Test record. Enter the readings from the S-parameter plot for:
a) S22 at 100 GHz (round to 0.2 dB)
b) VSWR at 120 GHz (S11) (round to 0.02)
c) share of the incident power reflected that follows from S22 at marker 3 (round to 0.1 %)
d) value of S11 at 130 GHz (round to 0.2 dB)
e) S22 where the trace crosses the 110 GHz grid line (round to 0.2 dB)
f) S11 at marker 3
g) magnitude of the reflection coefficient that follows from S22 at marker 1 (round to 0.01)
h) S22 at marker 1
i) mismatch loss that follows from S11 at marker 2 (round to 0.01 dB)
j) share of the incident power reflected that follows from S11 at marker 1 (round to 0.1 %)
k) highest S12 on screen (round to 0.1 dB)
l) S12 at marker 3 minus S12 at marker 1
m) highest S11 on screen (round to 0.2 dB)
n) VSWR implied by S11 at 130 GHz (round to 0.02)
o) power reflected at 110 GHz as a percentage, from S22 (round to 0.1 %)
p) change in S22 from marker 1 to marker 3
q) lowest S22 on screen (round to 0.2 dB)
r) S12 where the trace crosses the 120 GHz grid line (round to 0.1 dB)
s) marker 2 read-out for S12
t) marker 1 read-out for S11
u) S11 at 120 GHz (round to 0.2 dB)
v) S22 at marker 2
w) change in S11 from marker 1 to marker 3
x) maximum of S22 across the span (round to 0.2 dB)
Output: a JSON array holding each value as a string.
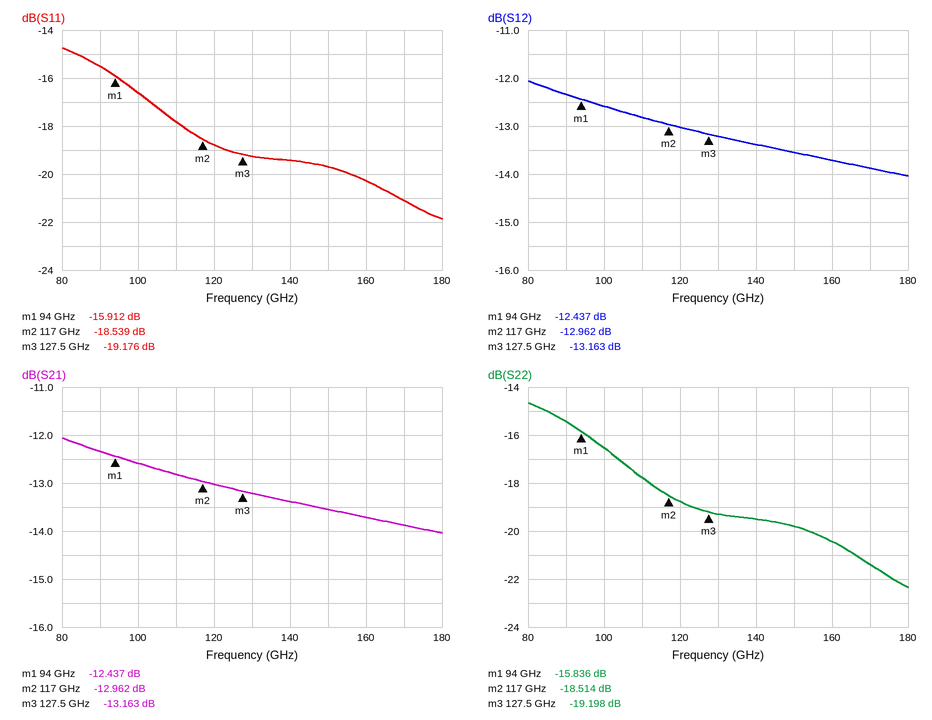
["-16.6 dB", "1.26", "1.2 %", "-19.2 dB", "-17.8 dB", "-19.176 dB", "0.16", "-15.836 dB", "0.06 dB", "2.6 %", "-12.1 dB", "-0.726 dB", "-14.8 dB", "1.24", "1.7 %", "-3.362 dB", "-22.4 dB", "-13.0 dB", "-12.962 dB", "-15.912 dB", "-18.8 dB", "-18.514 dB", "-3.264 dB", "-14.6 dB"]
